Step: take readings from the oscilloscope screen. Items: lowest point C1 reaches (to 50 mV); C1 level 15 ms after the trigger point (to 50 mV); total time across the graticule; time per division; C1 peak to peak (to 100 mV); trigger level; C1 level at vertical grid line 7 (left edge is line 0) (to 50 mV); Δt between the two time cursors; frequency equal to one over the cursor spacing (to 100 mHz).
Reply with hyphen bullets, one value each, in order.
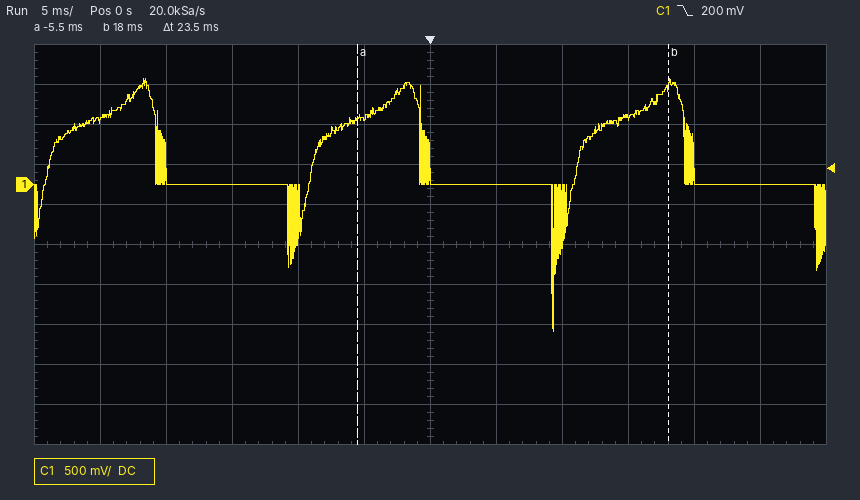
- -1.85 V
- 850 mV
- 60 ms
- 5 ms
- 3.20 V
- 200 mV
- 0 mV
- 23.5 ms
- 42.6 Hz
